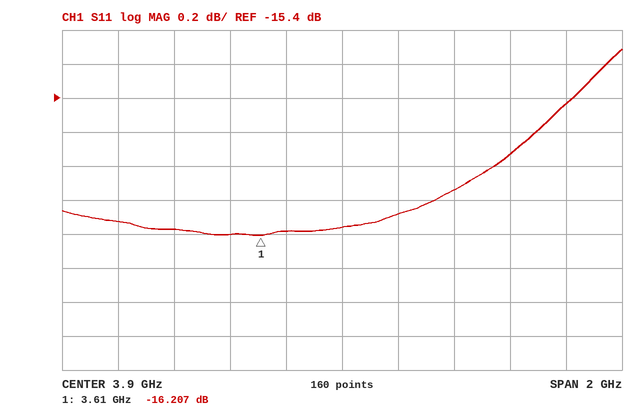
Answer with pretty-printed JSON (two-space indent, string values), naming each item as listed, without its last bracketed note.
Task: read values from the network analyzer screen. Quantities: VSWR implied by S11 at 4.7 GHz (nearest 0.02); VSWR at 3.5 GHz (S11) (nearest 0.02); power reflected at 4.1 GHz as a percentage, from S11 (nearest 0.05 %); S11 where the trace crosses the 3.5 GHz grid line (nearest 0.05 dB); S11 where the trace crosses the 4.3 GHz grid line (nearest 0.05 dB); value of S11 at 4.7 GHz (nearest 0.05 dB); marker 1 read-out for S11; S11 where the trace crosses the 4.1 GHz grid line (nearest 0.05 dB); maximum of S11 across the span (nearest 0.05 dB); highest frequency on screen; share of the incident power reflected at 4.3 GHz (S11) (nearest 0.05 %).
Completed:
{
  "VSWR implied by S11 at 4.7 GHz": "1.40",
  "VSWR at 3.5 GHz (S11)": "1.36",
  "power reflected at 4.1 GHz as a percentage, from S11": "2.45 %",
  "S11 where the trace crosses the 3.5 GHz grid line": "-16.20 dB",
  "S11 where the trace crosses the 4.3 GHz grid line": "-15.95 dB",
  "value of S11 at 4.7 GHz": "-15.45 dB",
  "marker 1 read-out for S11": "-16.207 dB",
  "S11 where the trace crosses the 4.1 GHz grid line": "-16.10 dB",
  "maximum of S11 across the span": "-15.10 dB",
  "highest frequency on screen": "4.9 GHz",
  "share of the incident power reflected at 4.3 GHz (S11)": "2.55 %"
}
